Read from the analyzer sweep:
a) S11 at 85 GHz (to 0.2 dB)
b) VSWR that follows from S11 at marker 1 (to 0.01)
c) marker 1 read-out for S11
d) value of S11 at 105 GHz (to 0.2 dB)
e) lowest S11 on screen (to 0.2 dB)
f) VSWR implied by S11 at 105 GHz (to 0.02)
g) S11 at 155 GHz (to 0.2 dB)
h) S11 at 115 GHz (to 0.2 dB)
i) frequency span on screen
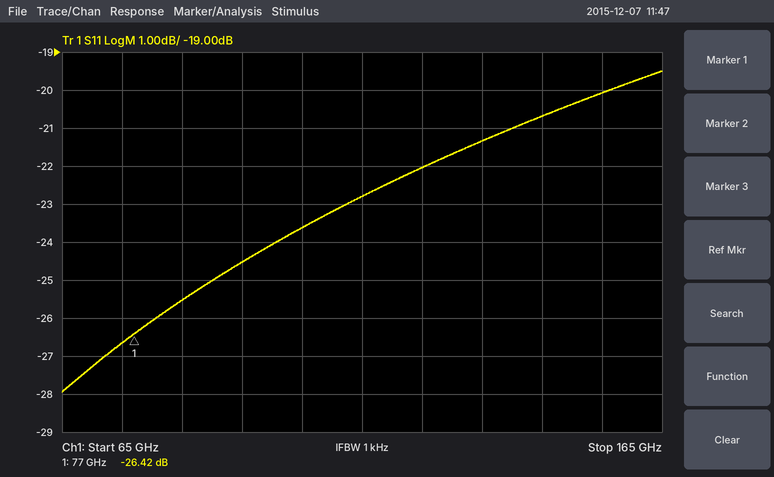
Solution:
-25.6 dB
1.10
-26.42 dB
-23.6 dB
-28.0 dB
1.14
-20.0 dB
-22.8 dB
100 GHz
